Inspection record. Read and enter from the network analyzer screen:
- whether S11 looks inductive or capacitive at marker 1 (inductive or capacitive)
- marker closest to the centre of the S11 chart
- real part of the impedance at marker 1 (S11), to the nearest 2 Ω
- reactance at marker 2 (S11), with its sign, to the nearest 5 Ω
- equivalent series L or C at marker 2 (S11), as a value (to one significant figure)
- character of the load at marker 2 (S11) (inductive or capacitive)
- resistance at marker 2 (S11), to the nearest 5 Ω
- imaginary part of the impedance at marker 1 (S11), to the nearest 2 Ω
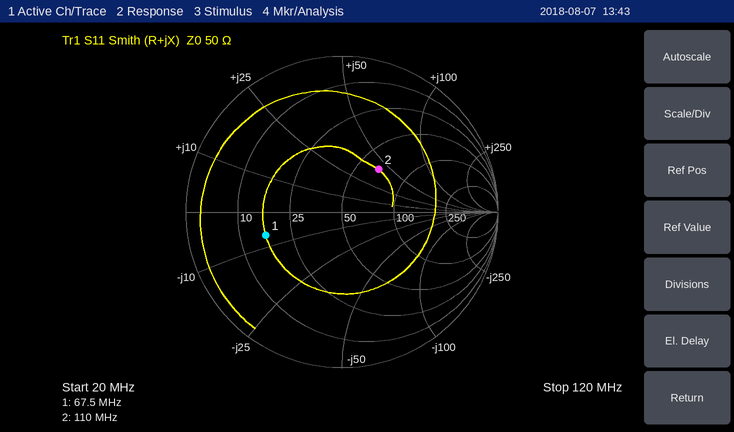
capacitive
marker 2
16 Ω
+40 Ω
60 nH
inductive
65 Ω
-6 Ω
